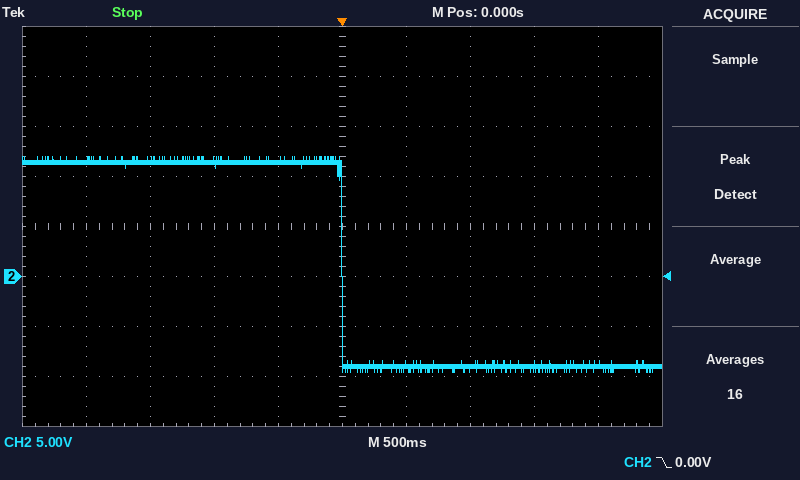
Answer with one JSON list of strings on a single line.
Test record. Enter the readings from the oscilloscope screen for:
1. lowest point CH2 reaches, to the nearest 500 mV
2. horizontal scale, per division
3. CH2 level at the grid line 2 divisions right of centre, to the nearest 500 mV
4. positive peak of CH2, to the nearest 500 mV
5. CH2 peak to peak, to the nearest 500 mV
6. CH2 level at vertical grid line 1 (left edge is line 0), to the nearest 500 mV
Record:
["-9.5 V", "500 ms", "-9.0 V", "12.0 V", "21.5 V", "11.5 V"]
